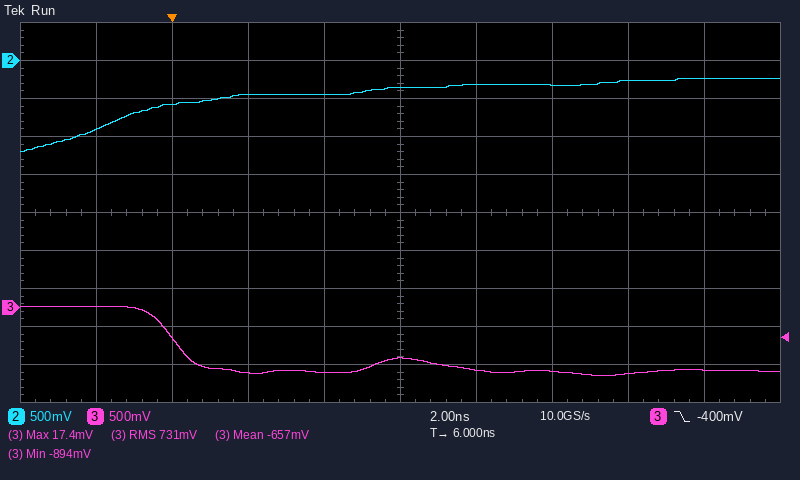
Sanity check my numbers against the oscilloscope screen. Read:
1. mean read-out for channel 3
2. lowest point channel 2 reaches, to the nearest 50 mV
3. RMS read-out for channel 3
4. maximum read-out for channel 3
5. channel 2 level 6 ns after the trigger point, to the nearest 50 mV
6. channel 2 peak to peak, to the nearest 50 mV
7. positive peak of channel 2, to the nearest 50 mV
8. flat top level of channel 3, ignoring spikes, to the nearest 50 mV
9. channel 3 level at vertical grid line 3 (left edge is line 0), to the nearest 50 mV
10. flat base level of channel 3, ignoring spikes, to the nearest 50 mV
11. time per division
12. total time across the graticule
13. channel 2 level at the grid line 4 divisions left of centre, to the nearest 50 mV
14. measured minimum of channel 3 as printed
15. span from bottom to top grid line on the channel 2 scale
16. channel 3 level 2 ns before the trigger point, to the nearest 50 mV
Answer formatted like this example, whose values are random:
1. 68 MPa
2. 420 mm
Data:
1. -657 mV
2. -1.20 V
3. 731 mV
4. 17.4 mV
5. -350 mV
6. 950 mV
7. -250 mV
8. 0 mV
9. -850 mV
10. -850 mV
11. 2 ns
12. 20 ns
13. -900 mV
14. -894 mV
15. 5 V
16. 0 mV
